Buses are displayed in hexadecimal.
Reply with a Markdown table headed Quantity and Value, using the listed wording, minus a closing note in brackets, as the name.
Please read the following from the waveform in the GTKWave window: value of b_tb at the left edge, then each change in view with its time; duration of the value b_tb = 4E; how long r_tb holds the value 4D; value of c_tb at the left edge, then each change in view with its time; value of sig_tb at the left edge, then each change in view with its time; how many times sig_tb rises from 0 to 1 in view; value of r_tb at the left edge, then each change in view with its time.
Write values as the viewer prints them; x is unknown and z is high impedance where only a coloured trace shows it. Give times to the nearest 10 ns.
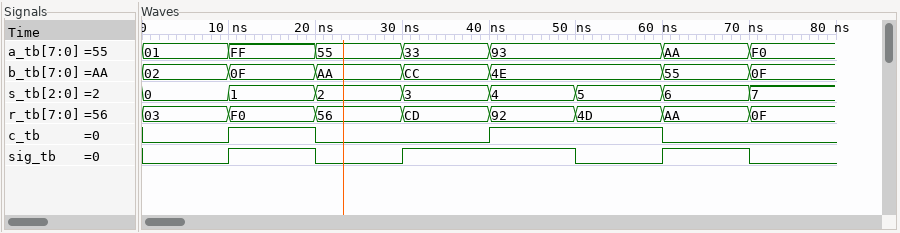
| Quantity | Value |
|---|---|
| value of b_tb at the left edge, then each change in view with its time | 02, 0F at 10 ns, AA at 20 ns, CC at 30 ns, 4E at 40 ns, 55 at 60 ns, 0F at 70 ns |
| duration of the value b_tb = 4E | 20 ns |
| how long r_tb holds the value 4D | 10 ns |
| value of c_tb at the left edge, then each change in view with its time | 0, 1 at 10 ns, 0 at 20 ns, 1 at 40 ns, 0 at 60 ns |
| value of sig_tb at the left edge, then each change in view with its time | 0, 1 at 10 ns, 0 at 20 ns, 1 at 30 ns, 0 at 50 ns, 1 at 60 ns, 0 at 70 ns |
| how many times sig_tb rises from 0 to 1 in view | 3 |
| value of r_tb at the left edge, then each change in view with its time | 03, F0 at 10 ns, 56 at 20 ns, CD at 30 ns, 92 at 40 ns, 4D at 50 ns, AA at 60 ns, 0F at 70 ns |
